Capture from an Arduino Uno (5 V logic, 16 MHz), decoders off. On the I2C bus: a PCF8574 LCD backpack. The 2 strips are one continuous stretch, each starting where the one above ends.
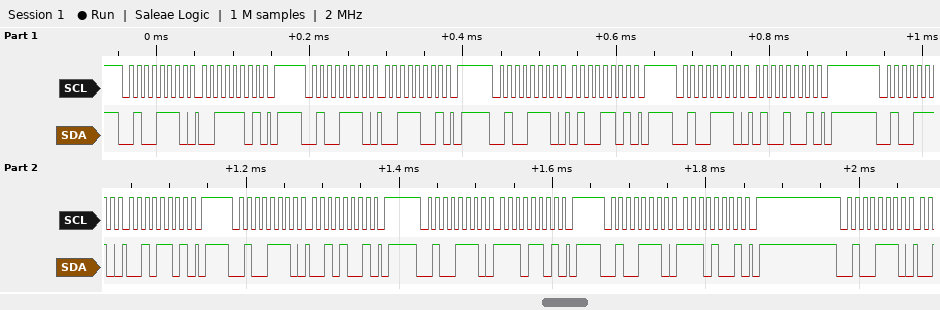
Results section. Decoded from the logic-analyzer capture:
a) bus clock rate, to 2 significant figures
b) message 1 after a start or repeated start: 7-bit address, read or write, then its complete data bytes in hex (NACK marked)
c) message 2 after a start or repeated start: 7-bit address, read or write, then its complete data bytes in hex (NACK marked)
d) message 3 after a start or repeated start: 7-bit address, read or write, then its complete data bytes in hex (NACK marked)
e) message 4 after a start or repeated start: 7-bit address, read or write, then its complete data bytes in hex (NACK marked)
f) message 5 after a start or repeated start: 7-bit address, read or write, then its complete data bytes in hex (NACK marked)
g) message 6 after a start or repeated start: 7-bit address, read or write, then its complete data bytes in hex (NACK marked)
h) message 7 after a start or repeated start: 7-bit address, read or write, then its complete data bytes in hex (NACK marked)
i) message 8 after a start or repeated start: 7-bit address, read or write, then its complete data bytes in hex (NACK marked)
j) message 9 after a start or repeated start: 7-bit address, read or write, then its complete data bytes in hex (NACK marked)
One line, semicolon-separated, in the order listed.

100 kHz; 0x27 write: 3D; 0x27 write: 39; 0x27 write: 4D; 0x27 write: 49; 0x27 write: 2D; 0x27 write: 29; 0x27 write: ED; 0x27 write: E9; 0x27 write
